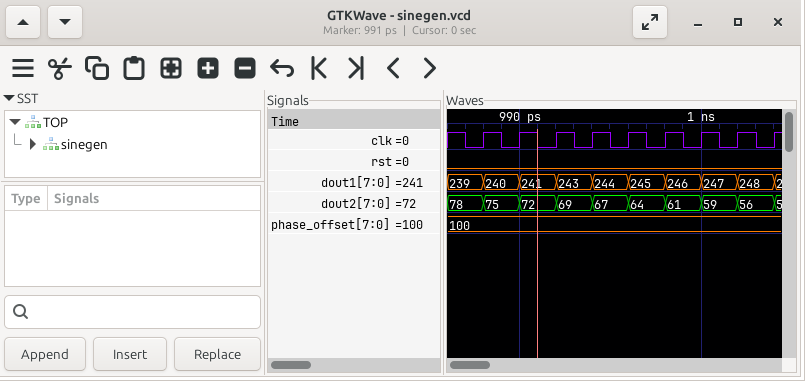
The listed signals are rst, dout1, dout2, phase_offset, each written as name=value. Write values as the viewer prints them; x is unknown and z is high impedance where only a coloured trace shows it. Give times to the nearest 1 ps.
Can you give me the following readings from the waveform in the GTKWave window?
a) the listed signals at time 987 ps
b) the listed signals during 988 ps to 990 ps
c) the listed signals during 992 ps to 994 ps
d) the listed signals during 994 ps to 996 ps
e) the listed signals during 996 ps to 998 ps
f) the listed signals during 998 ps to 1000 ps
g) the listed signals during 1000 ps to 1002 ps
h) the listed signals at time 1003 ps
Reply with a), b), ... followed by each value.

a) rst=0, dout1=239, dout2=78, phase_offset=100
b) rst=0, dout1=240, dout2=75, phase_offset=100
c) rst=0, dout1=243, dout2=69, phase_offset=100
d) rst=0, dout1=244, dout2=67, phase_offset=100
e) rst=0, dout1=245, dout2=64, phase_offset=100
f) rst=0, dout1=246, dout2=61, phase_offset=100
g) rst=0, dout1=247, dout2=59, phase_offset=100
h) rst=0, dout1=248, dout2=56, phase_offset=100
